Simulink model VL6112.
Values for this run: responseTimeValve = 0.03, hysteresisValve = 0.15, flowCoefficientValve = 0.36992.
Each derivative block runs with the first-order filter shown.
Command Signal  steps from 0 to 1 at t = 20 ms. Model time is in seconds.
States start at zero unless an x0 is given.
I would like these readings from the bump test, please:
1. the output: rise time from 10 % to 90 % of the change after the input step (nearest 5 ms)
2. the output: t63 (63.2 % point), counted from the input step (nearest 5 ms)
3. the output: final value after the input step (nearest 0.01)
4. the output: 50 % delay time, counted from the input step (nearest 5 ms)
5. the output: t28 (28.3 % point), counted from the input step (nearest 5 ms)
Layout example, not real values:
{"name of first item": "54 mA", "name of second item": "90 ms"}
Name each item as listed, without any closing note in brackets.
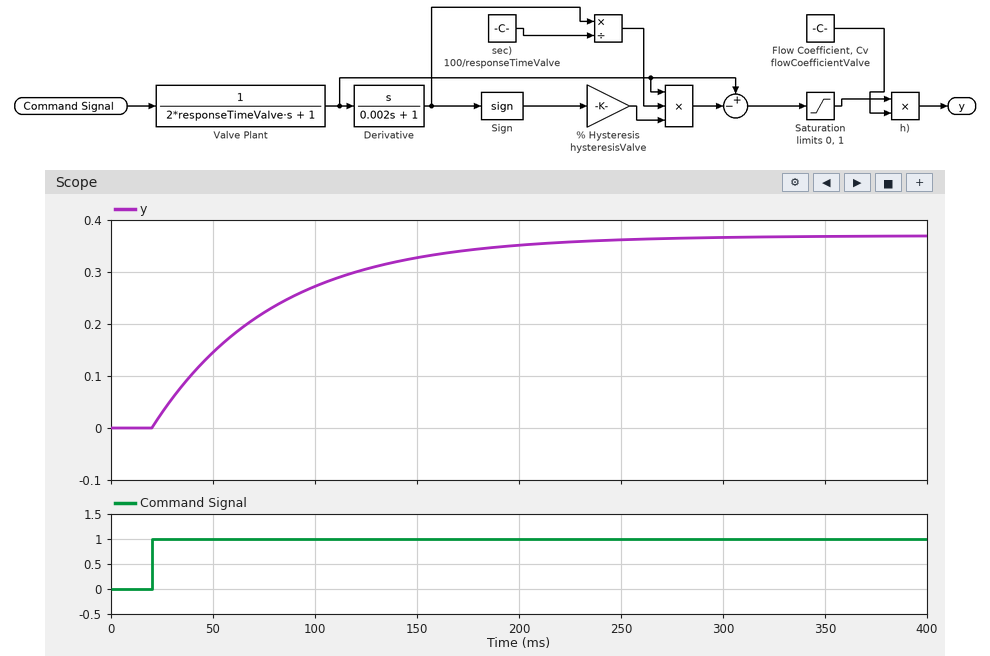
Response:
{"the output: rise time from 10 % to 90 % of the change after the input step": "130 ms", "the output: t63 (63.2 % point), counted from the input step": "60 ms", "the output: final value after the input step": "0.37", "the output: 50 % delay time, counted from the input step": "40 ms", "the output: t28 (28.3 % point), counted from the input step": "20 ms"}
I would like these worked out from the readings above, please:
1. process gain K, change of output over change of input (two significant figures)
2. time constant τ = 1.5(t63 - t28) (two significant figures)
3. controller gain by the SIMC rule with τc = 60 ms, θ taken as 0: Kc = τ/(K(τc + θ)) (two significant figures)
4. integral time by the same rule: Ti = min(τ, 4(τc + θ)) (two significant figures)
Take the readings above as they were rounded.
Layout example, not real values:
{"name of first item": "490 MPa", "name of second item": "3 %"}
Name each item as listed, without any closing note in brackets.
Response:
{"process gain K, change of output over change of input": "0.37", "time constant τ = 1.5(t63 - t28)": "60 ms", "controller gain by the SIMC rule with τc = 60 ms, θ taken as 0: Kc = τ/(K(τc + θ))": "2.7", "integral time by the same rule: Ti = min(τ, 4(τc + θ))": "60 ms"}
